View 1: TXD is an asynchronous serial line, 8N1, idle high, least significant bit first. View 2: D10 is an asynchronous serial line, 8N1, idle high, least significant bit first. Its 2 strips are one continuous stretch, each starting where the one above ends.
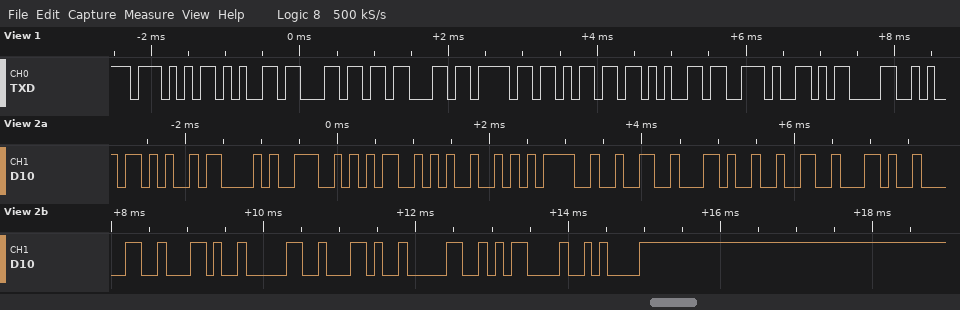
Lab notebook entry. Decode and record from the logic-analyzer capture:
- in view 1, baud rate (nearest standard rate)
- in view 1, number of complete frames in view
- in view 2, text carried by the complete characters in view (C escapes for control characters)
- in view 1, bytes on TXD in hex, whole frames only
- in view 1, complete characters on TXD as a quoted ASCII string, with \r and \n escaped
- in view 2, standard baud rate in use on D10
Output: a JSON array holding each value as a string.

["9600 baud", "9", "\"+CNMI=2,2,0,0,0\\r\\n\"", "57 65 6C 63 6F 6D 65 2E 0D", "\"Welcome.\\r\"", "9600 baud"]
